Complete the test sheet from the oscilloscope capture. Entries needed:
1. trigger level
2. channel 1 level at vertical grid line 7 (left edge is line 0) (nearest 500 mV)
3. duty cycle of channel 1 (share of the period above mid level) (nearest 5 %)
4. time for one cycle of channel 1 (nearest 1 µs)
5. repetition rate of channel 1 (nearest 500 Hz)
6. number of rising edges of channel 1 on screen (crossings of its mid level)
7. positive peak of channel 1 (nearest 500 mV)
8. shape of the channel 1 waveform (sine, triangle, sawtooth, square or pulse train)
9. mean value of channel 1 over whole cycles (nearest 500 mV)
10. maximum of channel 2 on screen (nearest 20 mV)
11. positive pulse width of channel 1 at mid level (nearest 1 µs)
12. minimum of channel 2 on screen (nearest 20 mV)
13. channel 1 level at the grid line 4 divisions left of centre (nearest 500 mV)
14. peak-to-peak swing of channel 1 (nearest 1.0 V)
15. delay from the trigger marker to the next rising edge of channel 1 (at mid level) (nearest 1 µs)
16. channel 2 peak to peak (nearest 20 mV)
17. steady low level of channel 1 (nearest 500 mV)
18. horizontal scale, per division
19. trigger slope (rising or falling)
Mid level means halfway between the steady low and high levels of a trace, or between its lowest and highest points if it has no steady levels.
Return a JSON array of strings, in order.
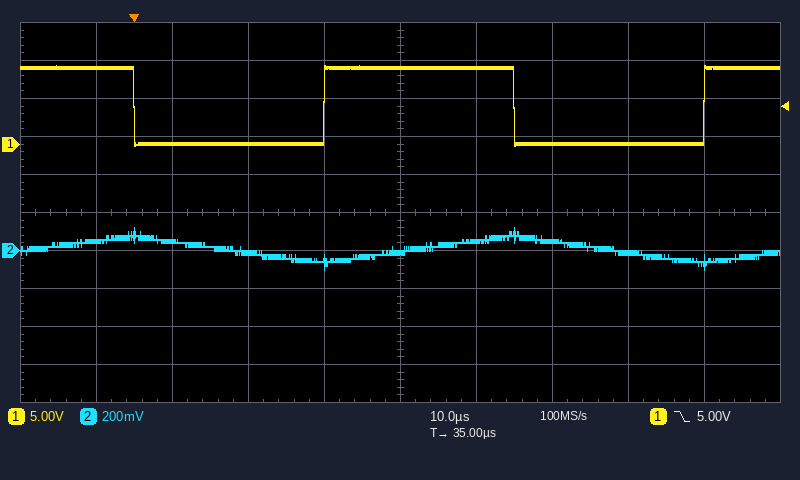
["5.00 V", "0.0 V", "50 %", "50 µs", "20.0 kHz", "2", "10.5 V", "square", "5.0 V", "120 mV", "25 µs", "-100 mV", "10.0 V", "11.0 V", "25 µs", "220 mV", "0.0 V", "10 µs", "falling"]
